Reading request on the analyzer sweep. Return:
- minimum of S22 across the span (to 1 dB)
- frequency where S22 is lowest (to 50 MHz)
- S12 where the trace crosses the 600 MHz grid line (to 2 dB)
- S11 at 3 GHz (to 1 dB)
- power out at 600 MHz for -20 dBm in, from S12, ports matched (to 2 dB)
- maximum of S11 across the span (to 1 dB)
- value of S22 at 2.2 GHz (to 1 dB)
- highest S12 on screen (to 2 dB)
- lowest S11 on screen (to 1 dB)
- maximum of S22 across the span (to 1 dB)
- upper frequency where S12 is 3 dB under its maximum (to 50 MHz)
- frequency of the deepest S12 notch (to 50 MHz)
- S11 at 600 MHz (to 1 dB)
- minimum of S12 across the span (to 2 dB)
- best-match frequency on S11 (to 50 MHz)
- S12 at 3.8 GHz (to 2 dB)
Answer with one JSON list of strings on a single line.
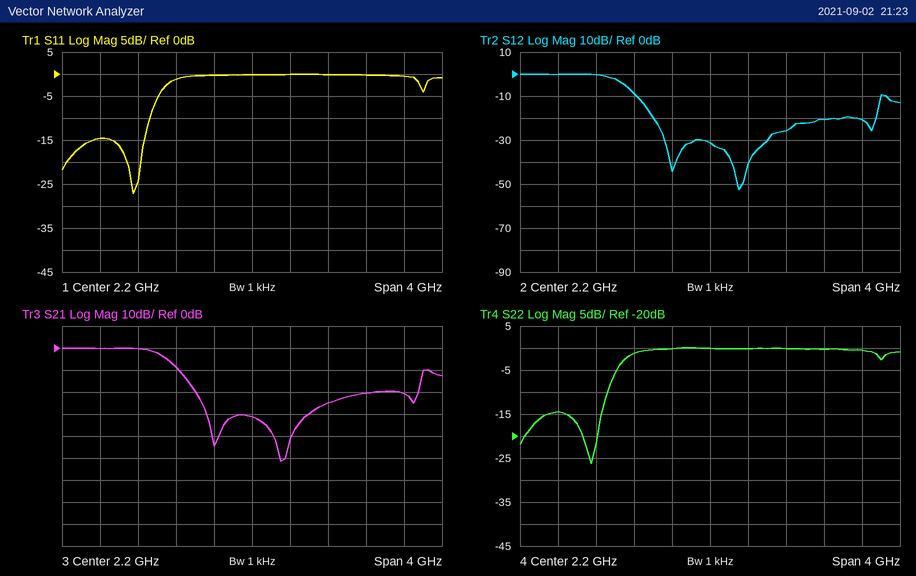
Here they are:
["-26 dB", "950 MHz", "0 dB", "0 dB", "-20 dBm", "0 dB", "0 dB", "0 dB", "-27 dB", "0 dB", "1.25 GHz", "2.50 GHz", "-15 dB", "-52 dB", "950 MHz", "-20 dB"]
